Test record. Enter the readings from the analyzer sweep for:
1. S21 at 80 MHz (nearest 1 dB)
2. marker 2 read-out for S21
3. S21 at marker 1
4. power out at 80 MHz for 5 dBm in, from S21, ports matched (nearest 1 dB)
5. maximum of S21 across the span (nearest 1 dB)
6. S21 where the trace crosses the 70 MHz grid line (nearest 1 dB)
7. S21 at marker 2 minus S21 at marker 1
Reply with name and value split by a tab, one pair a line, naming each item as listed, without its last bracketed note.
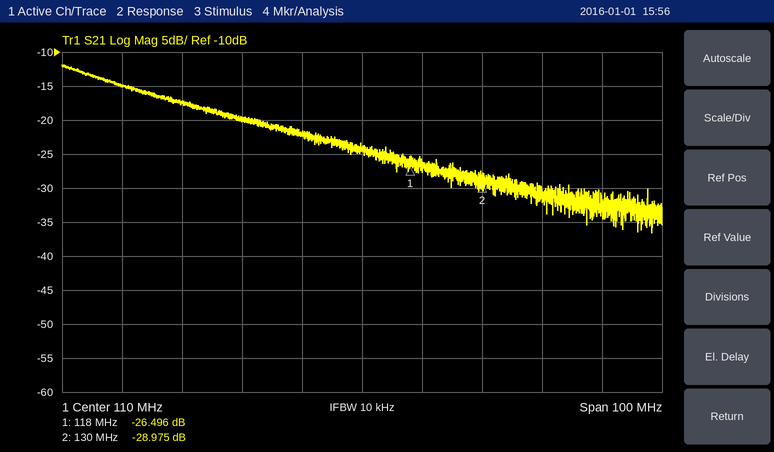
S21 at 80 MHz	-17 dB
marker 2 read-out for S21	-28.975 dB
S21 at marker 1	-26.496 dB
power out at 80 MHz for 5 dBm in, from S21, ports matched	-12 dBm
maximum of S21 across the span	-12 dB
S21 where the trace crosses the 70 MHz grid line	-15 dB
S21 at marker 2 minus S21 at marker 1	-2.479 dB
